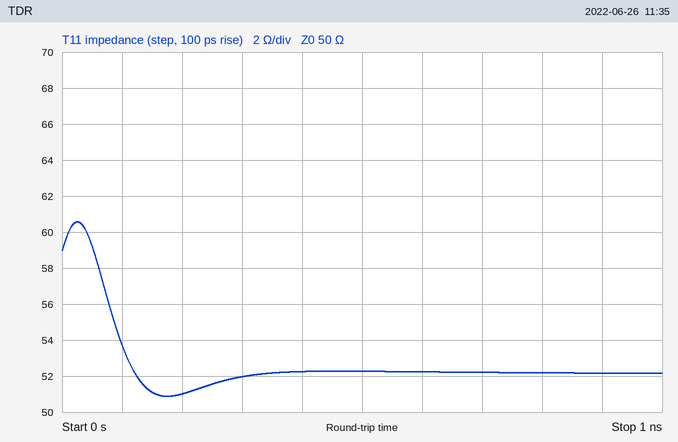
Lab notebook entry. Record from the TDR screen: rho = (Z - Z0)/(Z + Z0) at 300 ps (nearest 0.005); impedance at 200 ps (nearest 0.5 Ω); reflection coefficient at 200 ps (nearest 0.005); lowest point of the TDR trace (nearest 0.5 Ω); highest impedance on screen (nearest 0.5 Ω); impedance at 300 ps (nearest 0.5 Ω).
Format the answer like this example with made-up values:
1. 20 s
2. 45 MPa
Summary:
1. +0.020
2. 51.0 Ω
3. +0.010
4. 51.0 Ω
5. 60.5 Ω
6. 52.0 Ω
